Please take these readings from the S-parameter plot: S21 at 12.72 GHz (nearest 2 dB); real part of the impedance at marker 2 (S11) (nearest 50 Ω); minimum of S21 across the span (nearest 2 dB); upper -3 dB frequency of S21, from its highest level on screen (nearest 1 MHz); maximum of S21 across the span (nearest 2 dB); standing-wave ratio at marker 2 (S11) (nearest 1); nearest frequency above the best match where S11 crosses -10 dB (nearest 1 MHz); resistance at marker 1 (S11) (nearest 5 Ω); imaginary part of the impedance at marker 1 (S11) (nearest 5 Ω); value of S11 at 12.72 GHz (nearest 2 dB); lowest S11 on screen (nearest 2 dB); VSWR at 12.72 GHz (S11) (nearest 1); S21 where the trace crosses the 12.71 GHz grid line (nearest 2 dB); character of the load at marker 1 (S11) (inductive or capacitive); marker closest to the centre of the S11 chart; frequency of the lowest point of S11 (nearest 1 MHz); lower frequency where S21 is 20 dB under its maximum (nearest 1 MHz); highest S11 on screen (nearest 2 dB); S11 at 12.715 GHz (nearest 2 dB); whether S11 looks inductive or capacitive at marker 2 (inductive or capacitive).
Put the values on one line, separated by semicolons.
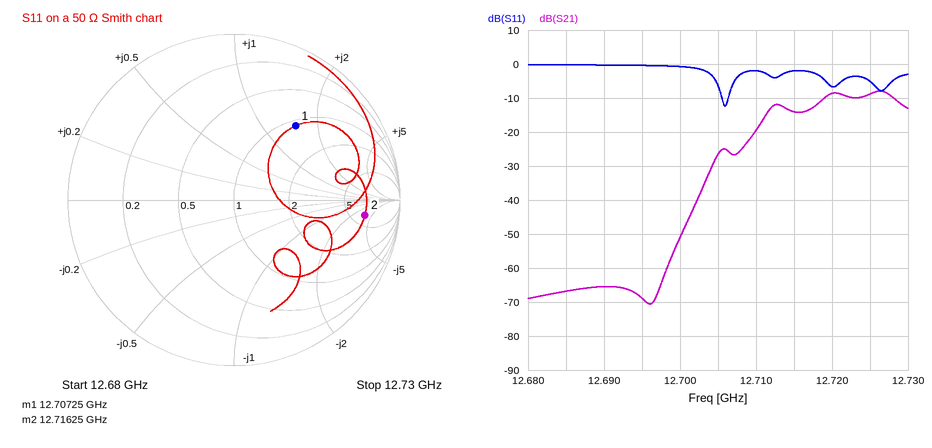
-8 dB; 350 Ω; -70 dB; 12.729 GHz; -8 dB; 9; 12.706 GHz; 55 Ω; +75 Ω; -6 dB; -12 dB; 3; -20 dB; inductive; marker 1; 12.706 GHz; 12.705 GHz; 0 dB; -2 dB; capacitive
